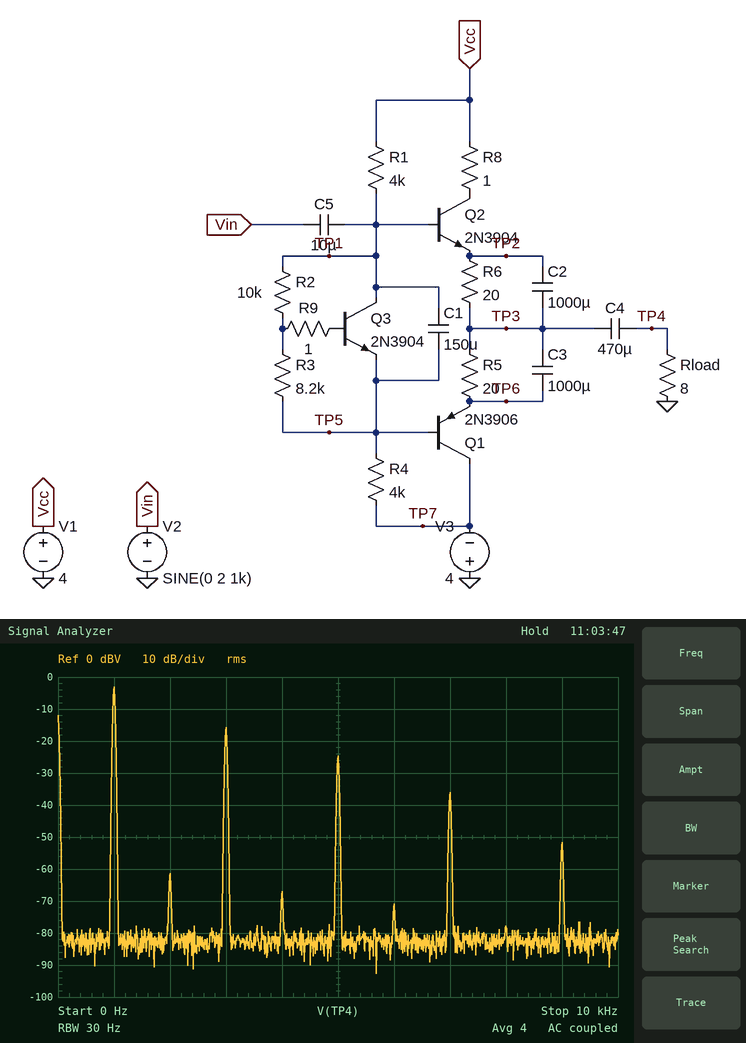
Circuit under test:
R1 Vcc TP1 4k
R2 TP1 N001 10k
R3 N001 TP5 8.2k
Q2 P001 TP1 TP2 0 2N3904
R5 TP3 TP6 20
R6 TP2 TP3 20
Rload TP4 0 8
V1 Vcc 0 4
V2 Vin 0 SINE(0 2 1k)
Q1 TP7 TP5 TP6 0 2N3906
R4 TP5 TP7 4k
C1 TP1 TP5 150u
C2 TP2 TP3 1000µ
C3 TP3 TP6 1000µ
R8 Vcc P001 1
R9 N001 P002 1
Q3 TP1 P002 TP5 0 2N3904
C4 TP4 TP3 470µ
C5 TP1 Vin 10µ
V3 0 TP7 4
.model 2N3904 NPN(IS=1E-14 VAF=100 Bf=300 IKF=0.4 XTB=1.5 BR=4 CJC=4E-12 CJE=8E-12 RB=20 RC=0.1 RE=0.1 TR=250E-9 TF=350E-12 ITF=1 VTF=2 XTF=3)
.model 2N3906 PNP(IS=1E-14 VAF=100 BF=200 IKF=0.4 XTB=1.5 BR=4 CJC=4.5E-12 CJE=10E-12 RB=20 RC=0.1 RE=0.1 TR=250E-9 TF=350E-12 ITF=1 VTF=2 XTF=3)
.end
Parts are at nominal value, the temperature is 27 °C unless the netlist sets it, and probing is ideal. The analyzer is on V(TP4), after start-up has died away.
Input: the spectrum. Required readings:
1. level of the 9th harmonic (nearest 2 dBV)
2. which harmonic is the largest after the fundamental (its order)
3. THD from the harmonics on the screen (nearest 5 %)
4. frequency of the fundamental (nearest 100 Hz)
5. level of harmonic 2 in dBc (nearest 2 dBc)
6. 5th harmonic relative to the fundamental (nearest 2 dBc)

-52 dBV
3
25 %
1.0 kHz
-58 dBc
-22 dBc
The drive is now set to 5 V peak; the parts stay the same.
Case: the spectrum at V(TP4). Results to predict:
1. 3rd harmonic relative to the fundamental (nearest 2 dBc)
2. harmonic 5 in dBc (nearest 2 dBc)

-10 dBc
-20 dBc
